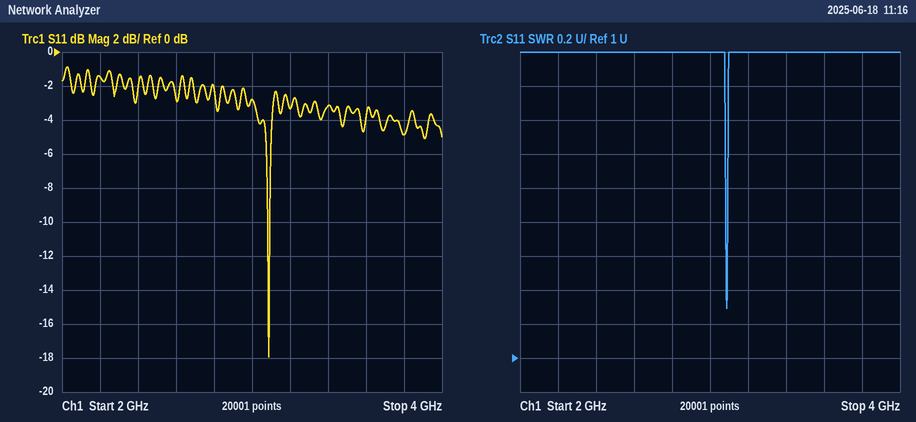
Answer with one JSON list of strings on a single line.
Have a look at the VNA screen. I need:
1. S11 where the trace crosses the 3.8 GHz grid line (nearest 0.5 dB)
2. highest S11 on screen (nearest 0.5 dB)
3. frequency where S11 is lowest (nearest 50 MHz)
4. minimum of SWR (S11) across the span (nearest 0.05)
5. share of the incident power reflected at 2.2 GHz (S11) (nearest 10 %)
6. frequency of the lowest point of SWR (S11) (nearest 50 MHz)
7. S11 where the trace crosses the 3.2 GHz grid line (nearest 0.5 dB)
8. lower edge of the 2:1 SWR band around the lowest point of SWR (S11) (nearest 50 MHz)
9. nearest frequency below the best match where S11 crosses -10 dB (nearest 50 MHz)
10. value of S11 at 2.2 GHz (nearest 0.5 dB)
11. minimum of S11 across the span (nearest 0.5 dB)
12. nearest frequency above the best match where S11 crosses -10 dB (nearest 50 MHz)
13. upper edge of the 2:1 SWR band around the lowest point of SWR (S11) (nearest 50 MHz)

["-5.0 dB", "-1.0 dB", "3.10 GHz", "1.30", "70 %", "3.10 GHz", "-3.5 dB", "3.10 GHz", "3.10 GHz", "-1.5 dB", "-18.0 dB", "3.10 GHz", "3.10 GHz"]
